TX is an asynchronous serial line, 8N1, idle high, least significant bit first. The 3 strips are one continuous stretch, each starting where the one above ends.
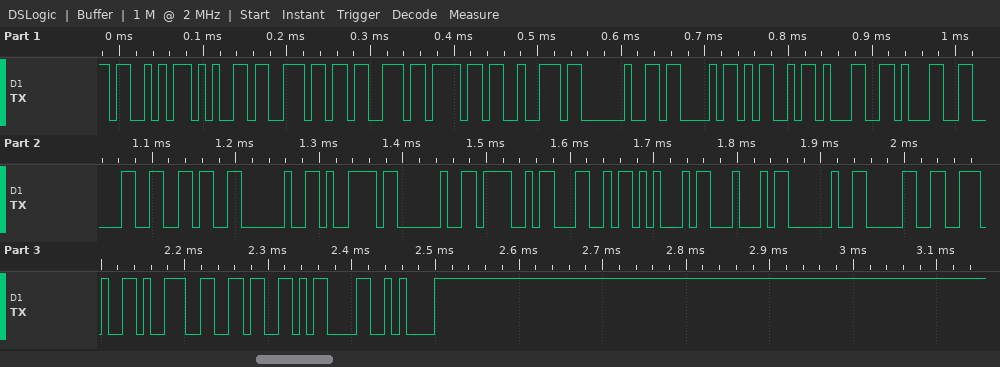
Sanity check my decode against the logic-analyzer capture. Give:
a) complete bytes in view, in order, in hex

53 65 6E 73 6F 72 20 43 4D 31 31 30 36 20 79 20 4F 4C 45 44 20 30 2E 39 36 0D 0A
